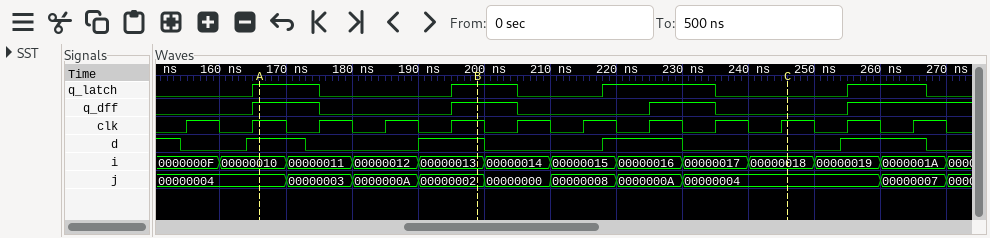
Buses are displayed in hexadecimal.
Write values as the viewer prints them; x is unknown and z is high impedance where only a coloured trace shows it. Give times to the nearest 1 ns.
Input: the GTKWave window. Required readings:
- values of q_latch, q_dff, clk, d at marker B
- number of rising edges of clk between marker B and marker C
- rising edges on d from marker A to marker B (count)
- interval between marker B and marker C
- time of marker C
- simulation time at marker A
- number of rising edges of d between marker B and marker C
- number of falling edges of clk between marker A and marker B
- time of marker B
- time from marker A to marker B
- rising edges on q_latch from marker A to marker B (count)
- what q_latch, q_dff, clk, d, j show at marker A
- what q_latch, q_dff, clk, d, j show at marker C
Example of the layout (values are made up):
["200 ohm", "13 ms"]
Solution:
["q_latch=1, q_dff=1, clk=1, d=1", "5", "1", "47 ns", "246 ns", "166 ns", "1", "3", "199 ns", "33 ns", "1", "q_latch=1, q_dff=1, clk=1, d=1, j=00000004", "q_latch=0, q_dff=0, clk=1, d=0, j=00000004"]
